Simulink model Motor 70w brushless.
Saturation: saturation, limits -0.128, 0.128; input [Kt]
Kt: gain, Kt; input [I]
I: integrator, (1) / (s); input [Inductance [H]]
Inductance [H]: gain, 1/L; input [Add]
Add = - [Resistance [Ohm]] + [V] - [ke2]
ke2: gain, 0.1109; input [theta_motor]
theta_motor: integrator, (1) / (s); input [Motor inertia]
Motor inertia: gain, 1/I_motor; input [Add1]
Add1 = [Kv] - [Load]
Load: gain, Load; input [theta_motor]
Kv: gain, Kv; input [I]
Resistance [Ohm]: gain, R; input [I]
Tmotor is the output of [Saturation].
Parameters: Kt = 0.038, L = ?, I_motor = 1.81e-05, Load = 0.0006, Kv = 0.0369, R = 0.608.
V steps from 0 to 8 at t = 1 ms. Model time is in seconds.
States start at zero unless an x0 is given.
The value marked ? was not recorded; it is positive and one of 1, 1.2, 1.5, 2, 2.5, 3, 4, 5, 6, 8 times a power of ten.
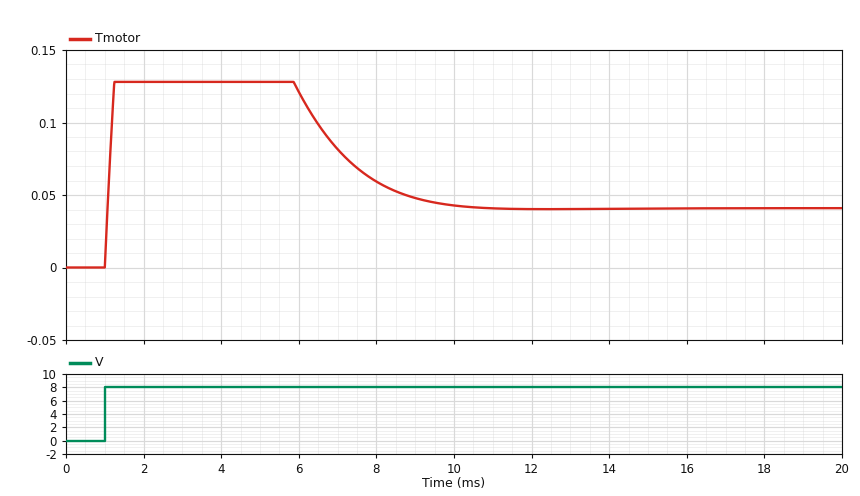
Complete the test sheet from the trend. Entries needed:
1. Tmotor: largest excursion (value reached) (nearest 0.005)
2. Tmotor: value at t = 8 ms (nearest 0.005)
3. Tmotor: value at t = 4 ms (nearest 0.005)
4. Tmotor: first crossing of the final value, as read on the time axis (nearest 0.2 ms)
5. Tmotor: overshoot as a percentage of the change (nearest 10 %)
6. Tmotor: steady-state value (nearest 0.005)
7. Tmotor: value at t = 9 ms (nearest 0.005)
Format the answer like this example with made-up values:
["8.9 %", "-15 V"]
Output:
["0.130", "0.060", "0.130", "1.0 ms", "210 %", "0.040", "0.050"]
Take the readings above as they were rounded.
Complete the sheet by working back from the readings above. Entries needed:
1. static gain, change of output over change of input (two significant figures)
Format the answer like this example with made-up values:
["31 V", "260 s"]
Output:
["0.0050"]
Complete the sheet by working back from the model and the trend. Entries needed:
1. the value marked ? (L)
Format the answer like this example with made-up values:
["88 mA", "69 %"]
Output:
["0.0005"]
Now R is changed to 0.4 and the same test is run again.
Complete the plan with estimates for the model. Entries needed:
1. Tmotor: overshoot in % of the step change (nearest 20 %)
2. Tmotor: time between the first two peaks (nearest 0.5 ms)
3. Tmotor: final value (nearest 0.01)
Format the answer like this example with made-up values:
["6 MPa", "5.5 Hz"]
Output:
["200 %", "10.5 ms", "0.04"]
